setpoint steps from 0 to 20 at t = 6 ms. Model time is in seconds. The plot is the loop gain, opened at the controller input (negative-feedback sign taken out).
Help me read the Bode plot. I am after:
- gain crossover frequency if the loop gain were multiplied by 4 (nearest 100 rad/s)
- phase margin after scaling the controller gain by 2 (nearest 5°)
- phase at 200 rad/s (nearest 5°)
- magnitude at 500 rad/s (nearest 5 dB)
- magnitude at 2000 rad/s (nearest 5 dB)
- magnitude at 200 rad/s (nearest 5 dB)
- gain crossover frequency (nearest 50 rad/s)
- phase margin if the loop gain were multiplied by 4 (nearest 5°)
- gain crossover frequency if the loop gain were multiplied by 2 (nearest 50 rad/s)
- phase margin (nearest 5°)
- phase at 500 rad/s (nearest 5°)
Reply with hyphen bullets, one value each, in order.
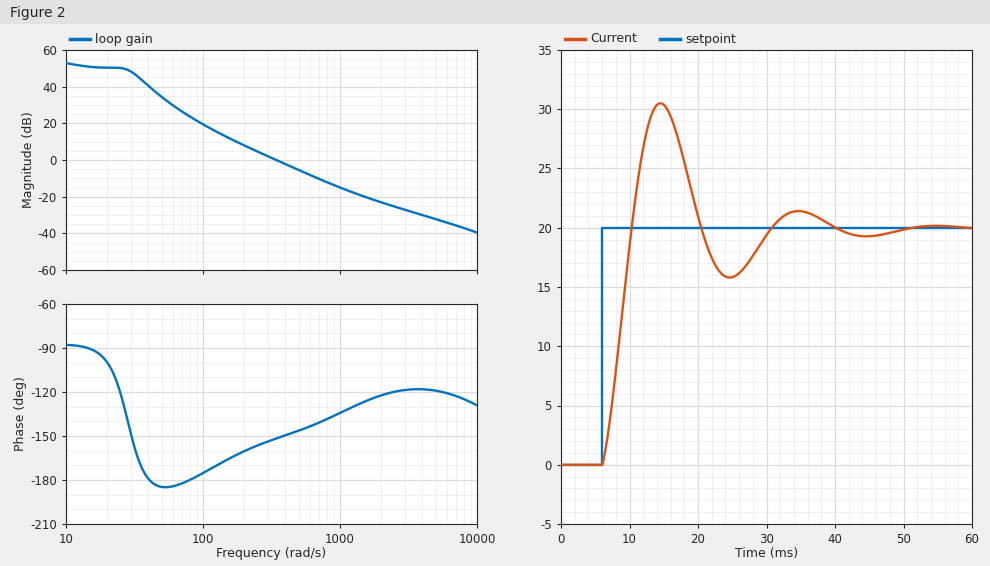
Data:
- 800 rad/s
- 35°
- -160°
- -5 dB
- -25 dB
- 10 dB
- 350 rad/s
- 40°
- 500 rad/s
- 30°
- -145°
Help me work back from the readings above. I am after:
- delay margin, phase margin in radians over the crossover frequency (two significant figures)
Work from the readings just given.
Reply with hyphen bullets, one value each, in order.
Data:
- 0.0015 s
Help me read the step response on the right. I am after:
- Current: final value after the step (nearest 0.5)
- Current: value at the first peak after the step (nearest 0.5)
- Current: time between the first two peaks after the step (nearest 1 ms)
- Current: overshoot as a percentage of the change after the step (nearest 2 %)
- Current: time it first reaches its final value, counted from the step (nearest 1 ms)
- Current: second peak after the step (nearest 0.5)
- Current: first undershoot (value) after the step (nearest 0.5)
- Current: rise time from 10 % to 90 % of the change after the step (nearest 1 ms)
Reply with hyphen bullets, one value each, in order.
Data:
- 20.0
- 30.5
- 20 ms
- 52 %
- 4 ms
- 21.5
- 16.0
- 3 ms
